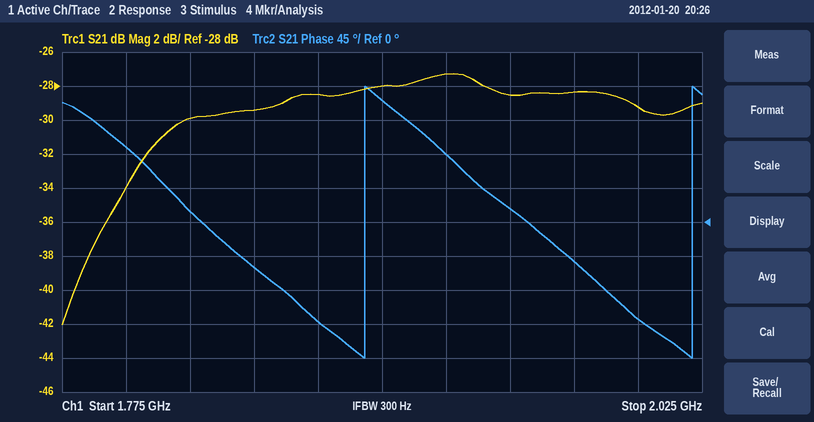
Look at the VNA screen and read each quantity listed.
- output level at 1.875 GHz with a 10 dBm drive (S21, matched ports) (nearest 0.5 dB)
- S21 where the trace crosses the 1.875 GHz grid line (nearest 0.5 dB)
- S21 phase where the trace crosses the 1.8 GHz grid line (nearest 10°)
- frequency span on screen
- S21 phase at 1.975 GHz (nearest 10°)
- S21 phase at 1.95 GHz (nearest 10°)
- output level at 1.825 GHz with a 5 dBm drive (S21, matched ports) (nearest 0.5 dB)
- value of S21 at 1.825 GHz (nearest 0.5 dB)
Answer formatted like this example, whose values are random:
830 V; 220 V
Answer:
-18.5 dBm; -28.5 dB; 100°; 250 MHz; -50°; 20°; -25.0 dBm; -30.0 dB
